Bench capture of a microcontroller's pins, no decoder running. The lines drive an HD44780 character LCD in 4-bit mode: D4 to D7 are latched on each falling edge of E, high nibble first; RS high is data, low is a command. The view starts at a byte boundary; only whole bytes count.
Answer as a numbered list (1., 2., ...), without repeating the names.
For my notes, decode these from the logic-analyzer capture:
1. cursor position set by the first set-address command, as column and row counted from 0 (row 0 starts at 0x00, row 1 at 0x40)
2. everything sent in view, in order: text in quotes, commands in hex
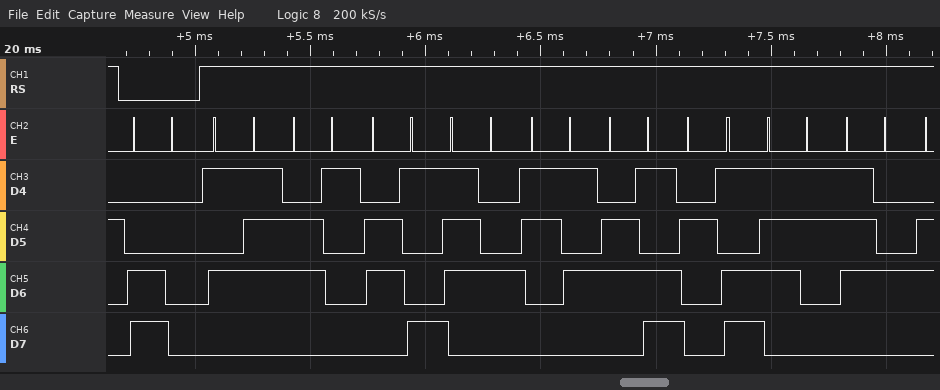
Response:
1. column 0, row 1
2. 0xC0 "Wait5m-st"
